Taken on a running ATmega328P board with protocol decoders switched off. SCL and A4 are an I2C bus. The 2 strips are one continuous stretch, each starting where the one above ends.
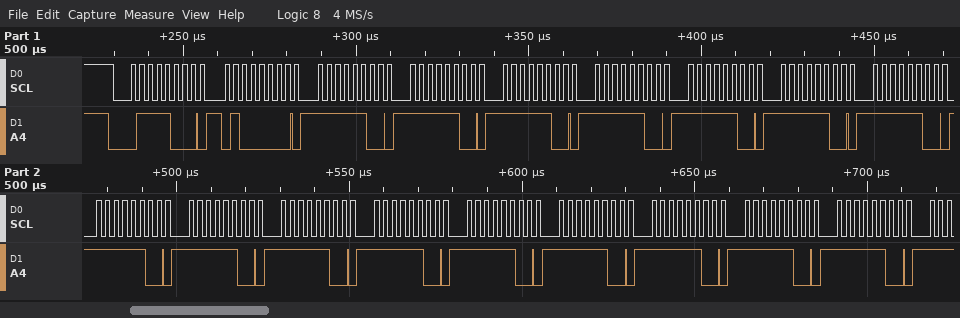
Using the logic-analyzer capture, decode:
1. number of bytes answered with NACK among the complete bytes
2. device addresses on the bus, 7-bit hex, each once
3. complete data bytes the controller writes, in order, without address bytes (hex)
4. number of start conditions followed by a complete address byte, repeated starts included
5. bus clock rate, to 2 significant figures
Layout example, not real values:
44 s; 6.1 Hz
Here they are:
0; 0x3C; 40 FC FC FC FC FC FC FC FC FC FC FC FC FC FC FC FC; 1; 400 kHz
